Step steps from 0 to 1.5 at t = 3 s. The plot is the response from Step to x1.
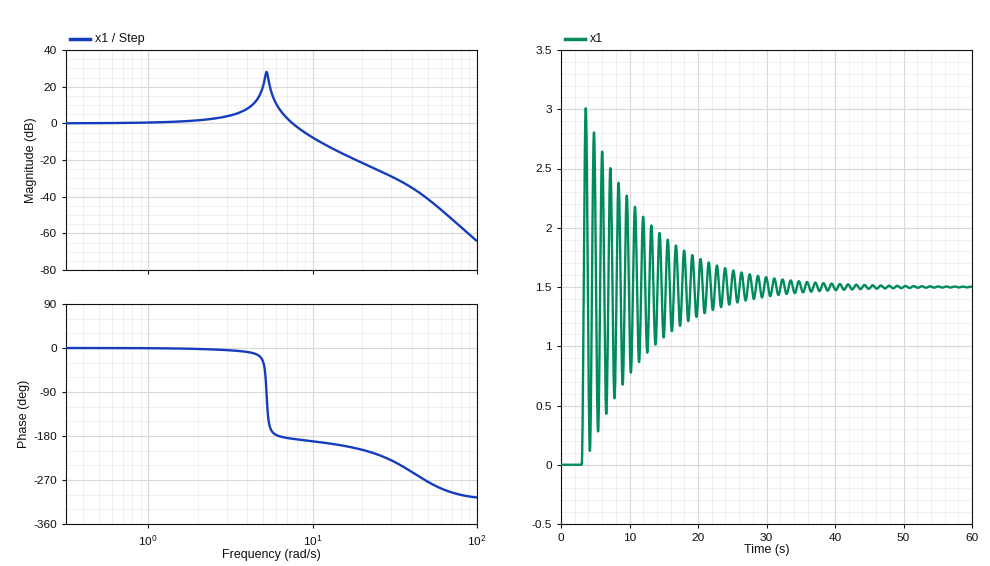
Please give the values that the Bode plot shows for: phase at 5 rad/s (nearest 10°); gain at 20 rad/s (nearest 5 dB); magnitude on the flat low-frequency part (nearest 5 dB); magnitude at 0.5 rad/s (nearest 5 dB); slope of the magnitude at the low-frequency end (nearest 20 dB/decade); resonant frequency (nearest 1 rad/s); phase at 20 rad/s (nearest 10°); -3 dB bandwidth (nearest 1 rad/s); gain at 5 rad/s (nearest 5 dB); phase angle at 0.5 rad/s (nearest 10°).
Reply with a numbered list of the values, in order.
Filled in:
1. -30°
2. -20 dB
3. 0 dB
4. 0 dB
5. 0 dB/decade
6. 5 rad/s
7. -210°
8. 8 rad/s
9. 20 dB
10. 0°
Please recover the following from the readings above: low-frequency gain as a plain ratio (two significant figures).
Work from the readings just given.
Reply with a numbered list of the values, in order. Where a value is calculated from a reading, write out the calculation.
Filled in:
1. 10^(0 / 20) = 1.0
